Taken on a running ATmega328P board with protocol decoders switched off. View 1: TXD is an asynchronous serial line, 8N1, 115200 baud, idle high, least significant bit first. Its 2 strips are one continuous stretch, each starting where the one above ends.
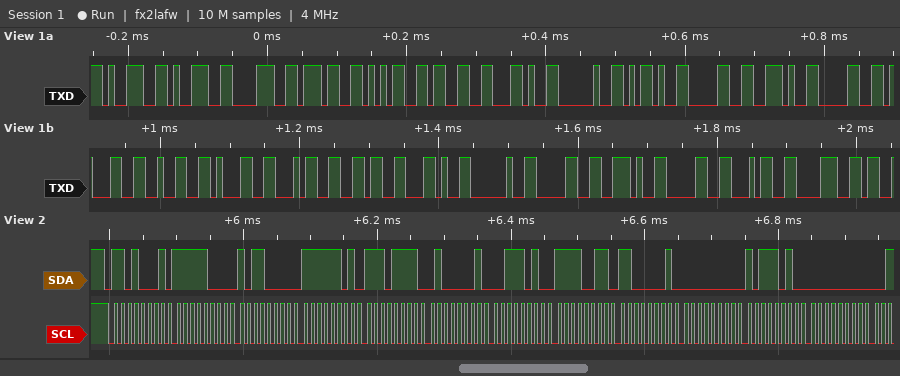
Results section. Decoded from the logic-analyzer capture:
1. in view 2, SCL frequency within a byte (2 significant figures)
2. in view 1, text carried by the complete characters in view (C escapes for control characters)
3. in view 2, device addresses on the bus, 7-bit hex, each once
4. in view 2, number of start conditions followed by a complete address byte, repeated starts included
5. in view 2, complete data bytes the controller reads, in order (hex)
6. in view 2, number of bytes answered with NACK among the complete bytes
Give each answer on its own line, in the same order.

100 kHz
"998753, -0.012146, 0.048"
0x68
1
F8 B0 FD EF 41 3A F3 C1 00 BA 00
0
